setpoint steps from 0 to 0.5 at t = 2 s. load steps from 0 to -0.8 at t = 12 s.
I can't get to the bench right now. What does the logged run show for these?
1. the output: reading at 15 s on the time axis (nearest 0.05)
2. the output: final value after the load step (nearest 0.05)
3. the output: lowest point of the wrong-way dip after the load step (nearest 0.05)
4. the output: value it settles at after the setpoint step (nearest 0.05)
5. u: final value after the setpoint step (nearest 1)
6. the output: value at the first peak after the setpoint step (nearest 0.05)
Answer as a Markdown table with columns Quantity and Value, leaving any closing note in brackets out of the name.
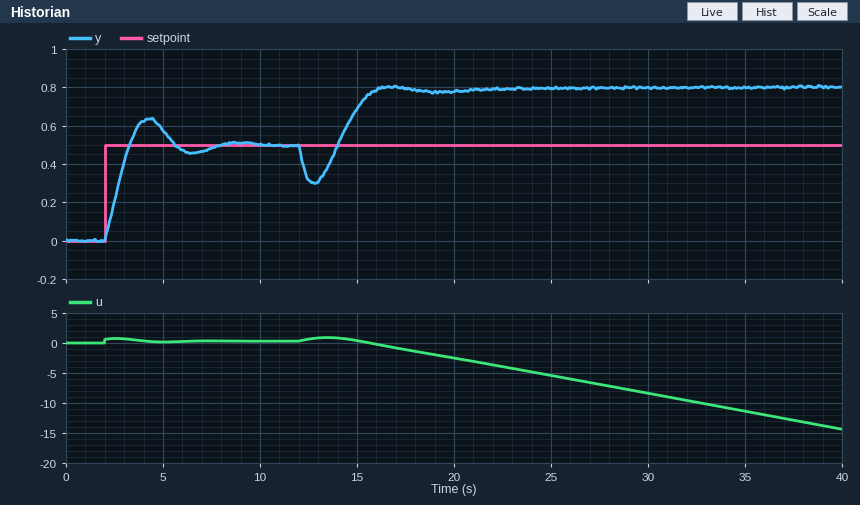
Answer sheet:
| Quantity | Value |
|---|---|
| the output: reading at 15 s on the time axis | 0.70 |
| the output: final value after the load step | 0.80 |
| the output: lowest point of the wrong-way dip after the load step | 0.30 |
| the output: value it settles at after the setpoint step | 0.50 |
| u: final value after the setpoint step | 0 |
| the output: value at the first peak after the setpoint step | 0.65 |
